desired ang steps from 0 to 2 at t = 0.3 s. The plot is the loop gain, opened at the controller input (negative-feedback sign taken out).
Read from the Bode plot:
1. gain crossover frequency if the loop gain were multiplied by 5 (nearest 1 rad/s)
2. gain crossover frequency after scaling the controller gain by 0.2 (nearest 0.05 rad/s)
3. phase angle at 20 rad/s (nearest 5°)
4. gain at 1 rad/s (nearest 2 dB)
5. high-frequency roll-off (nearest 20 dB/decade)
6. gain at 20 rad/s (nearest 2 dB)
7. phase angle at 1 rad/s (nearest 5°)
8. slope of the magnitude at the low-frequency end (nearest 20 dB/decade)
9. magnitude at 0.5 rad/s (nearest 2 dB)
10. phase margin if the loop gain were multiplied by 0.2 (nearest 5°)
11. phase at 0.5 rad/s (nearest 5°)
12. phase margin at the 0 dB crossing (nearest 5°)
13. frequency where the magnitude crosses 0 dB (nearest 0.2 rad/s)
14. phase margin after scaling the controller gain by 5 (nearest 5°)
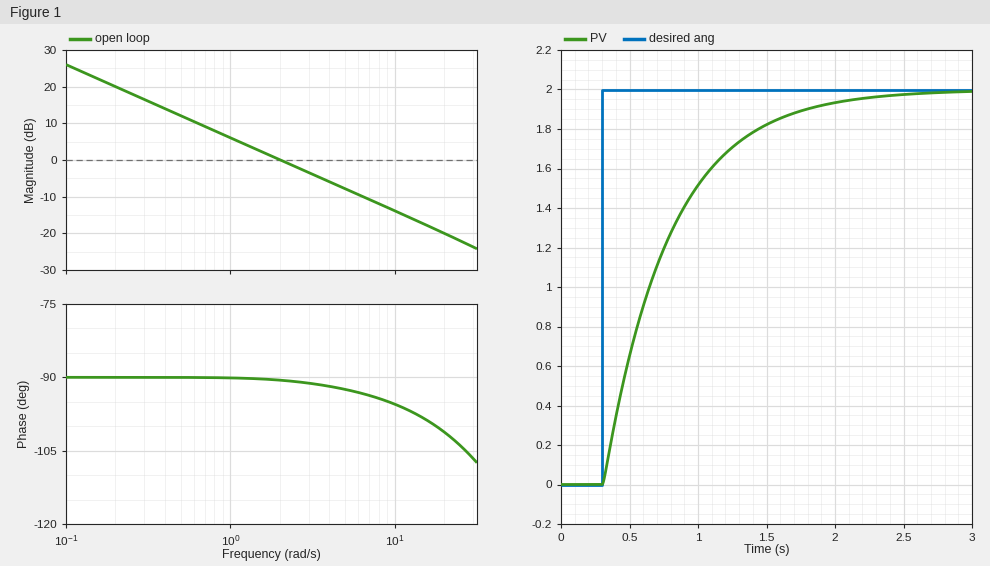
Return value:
10 rad/s
0.40 rad/s
-100°
6 dB
-20 dB/decade
-20 dB
-90°
-20 dB/decade
12 dB
90°
-90°
90°
2.0 rad/s
85°
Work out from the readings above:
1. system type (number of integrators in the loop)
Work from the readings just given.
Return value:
1
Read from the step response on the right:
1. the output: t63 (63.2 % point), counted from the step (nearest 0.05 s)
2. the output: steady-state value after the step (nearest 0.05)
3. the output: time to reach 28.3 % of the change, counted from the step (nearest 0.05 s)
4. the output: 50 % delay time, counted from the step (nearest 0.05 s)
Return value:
0.50 s
2.00
0.15 s
0.35 s
